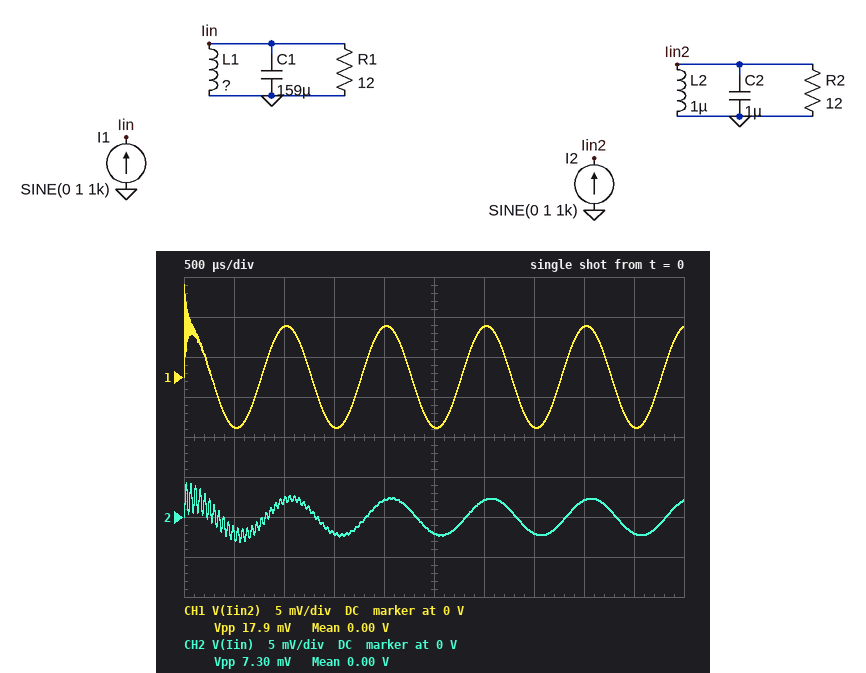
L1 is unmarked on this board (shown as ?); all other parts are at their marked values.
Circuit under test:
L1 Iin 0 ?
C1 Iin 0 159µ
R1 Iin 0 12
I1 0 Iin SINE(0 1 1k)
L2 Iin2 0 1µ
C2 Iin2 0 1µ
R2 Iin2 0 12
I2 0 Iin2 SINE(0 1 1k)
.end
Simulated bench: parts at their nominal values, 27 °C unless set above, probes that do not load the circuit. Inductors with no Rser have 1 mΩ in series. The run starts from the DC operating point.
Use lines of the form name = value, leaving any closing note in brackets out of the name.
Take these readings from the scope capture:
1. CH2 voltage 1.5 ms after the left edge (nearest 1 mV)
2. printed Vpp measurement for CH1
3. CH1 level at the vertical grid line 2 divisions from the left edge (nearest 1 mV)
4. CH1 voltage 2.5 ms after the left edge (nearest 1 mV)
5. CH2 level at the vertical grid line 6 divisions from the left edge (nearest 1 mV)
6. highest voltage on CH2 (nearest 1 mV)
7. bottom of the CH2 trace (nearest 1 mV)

CH2 voltage 1.5 ms after the left edge = -2 mV
printed Vpp measurement for CH1 = 17.9 mV
CH1 level at the vertical grid line 2 divisions from the left edge = 6 mV
CH1 voltage 2.5 ms after the left edge = -6 mV
CH2 level at the vertical grid line 6 divisions from the left edge = 2 mV
highest voltage on CH2 = 4 mV
bottom of the CH2 trace = -3 mV
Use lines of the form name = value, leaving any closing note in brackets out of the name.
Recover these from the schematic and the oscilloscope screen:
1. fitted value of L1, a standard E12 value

fitted value of L1, a standard E12 value = 330 nH
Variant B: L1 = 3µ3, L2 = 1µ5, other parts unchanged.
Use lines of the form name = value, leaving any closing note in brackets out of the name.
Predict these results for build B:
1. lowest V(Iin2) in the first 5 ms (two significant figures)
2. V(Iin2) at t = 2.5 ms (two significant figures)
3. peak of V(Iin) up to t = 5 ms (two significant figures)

lowest V(Iin2) in the first 5 ms = -9.5 mV
V(Iin2) at t = 2.5 ms = -9.4 mV
peak of V(Iin) up to t = 5 ms = 40 mV
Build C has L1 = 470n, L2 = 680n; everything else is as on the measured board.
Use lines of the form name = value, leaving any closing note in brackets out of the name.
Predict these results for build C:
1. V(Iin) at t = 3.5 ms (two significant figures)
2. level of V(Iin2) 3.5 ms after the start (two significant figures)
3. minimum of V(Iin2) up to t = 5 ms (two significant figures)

V(Iin) at t = 3.5 ms = -3.0 mV
level of V(Iin2) 3.5 ms after the start = -4.3 mV
minimum of V(Iin2) up to t = 5 ms = -4.4 mV
